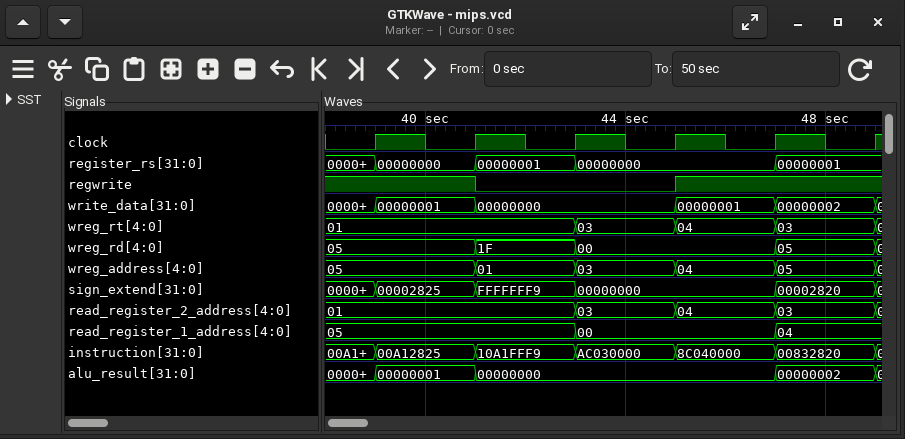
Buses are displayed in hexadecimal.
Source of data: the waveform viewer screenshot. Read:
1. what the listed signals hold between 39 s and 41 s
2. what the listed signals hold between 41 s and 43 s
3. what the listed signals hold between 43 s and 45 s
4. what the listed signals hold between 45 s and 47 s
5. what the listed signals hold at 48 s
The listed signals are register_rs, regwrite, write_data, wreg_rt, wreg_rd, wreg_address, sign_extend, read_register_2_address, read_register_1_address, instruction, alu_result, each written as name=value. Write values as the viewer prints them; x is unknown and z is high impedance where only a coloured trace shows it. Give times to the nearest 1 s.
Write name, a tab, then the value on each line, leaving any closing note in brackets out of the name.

what the listed signals hold between 39 s and 41 s	register_rs=00000000, regwrite=1, write_data=00000001, wreg_rt=01, wreg_rd=05, wreg_address=05, sign_extend=00002825, read_register_2_address=01, read_register_1_address=05, instruction=00A12825, alu_result=00000001
what the listed signals hold between 41 s and 43 s	register_rs=00000001, regwrite=0, write_data=00000000, wreg_rt=01, wreg_rd=1F, wreg_address=01, sign_extend=FFFFFFF9, read_register_2_address=01, read_register_1_address=05, instruction=10A1FFF9, alu_result=00000000
what the listed signals hold between 43 s and 45 s	register_rs=00000000, regwrite=0, write_data=00000000, wreg_rt=03, wreg_rd=00, wreg_address=03, sign_extend=00000000, read_register_2_address=03, read_register_1_address=00, instruction=AC030000, alu_result=00000000
what the listed signals hold between 45 s and 47 s	register_rs=00000000, regwrite=1, write_data=00000001, wreg_rt=04, wreg_rd=00, wreg_address=04, sign_extend=00000000, read_register_2_address=04, read_register_1_address=00, instruction=8C040000, alu_result=00000000
what the listed signals hold at 48 s	register_rs=00000001, regwrite=1, write_data=00000002, wreg_rt=03, wreg_rd=05, wreg_address=05, sign_extend=00002820, read_register_2_address=03, read_register_1_address=04, instruction=00832820, alu_result=00000002
